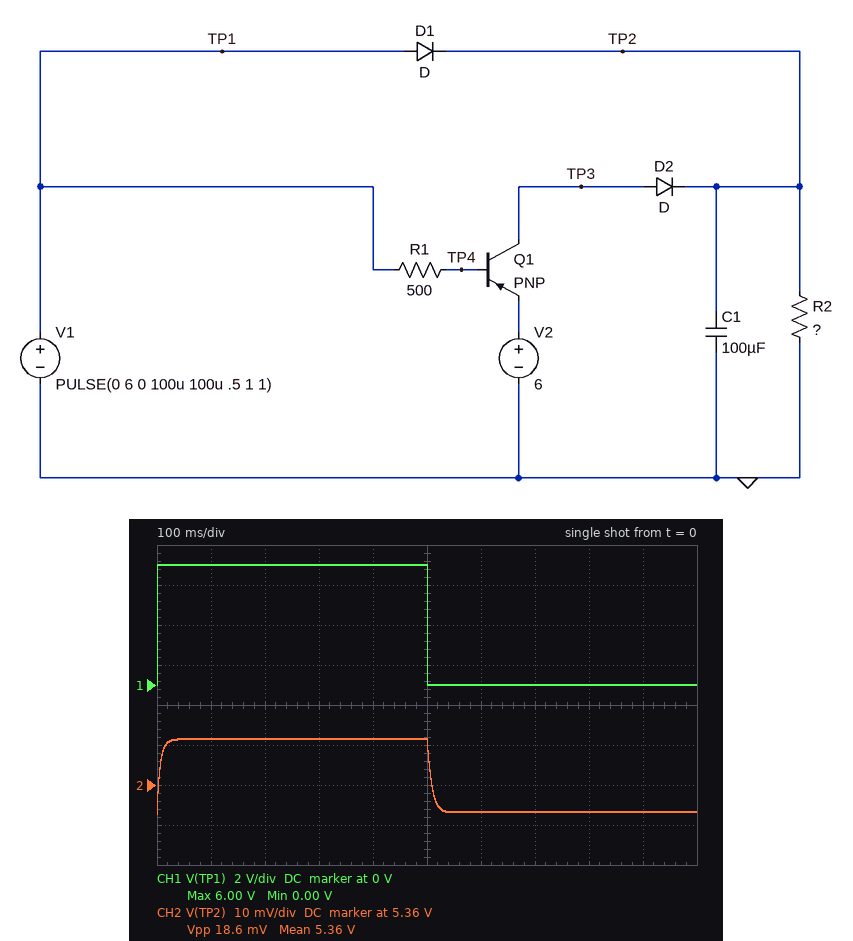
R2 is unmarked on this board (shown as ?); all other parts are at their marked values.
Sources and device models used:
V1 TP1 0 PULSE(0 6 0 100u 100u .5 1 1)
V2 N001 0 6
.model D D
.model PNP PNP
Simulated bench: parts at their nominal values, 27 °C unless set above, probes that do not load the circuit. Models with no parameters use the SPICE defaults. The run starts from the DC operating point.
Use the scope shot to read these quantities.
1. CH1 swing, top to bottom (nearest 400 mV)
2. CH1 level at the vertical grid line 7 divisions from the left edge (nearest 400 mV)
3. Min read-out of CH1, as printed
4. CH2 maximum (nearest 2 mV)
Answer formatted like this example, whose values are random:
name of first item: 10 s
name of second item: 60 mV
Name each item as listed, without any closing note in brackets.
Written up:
CH1 swing, top to bottom: 6.0 V
CH1 level at the vertical grid line 7 divisions from the left edge: 0 V
Min read-out of CH1, as printed: 0.00 V
CH2 maximum: 5.372 V
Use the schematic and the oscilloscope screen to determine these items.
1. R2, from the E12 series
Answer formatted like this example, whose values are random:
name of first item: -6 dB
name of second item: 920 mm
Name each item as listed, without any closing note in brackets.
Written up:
R2, from the E12 series: 15 kΩ
